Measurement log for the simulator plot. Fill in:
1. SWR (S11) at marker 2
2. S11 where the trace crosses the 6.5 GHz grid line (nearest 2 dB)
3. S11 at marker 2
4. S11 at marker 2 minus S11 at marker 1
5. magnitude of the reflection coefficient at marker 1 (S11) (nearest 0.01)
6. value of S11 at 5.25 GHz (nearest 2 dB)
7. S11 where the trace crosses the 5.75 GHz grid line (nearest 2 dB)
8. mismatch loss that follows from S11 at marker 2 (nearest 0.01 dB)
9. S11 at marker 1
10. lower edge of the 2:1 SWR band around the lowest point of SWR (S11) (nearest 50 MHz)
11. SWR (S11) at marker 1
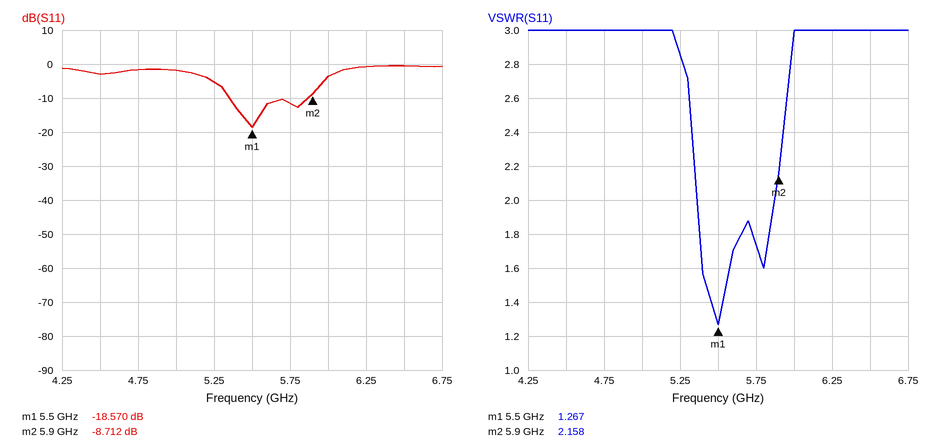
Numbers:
2.158
0 dB
-8.712 dB
9.858 dB
0.12
-6 dB
-12 dB
0.63 dB
-18.570 dB
5.35 GHz
1.267
